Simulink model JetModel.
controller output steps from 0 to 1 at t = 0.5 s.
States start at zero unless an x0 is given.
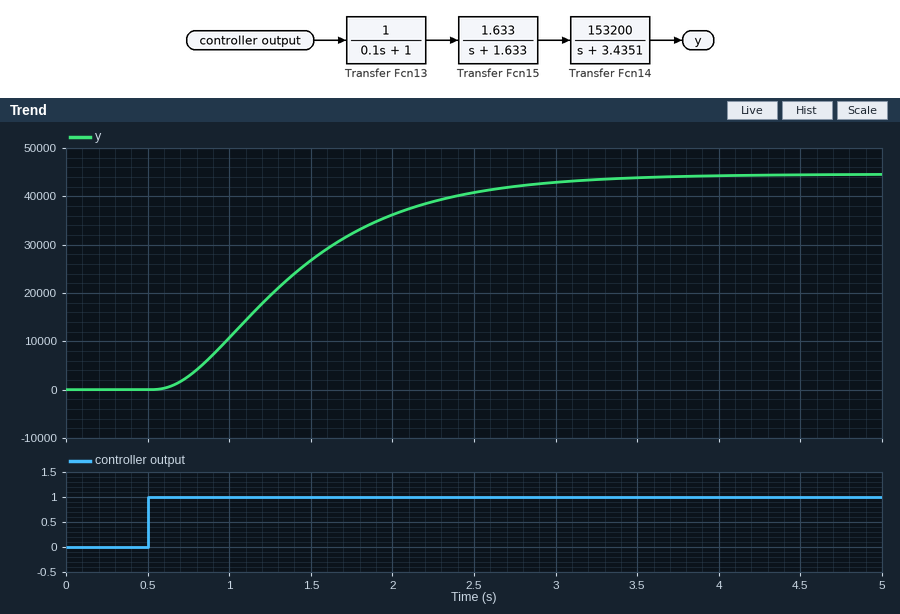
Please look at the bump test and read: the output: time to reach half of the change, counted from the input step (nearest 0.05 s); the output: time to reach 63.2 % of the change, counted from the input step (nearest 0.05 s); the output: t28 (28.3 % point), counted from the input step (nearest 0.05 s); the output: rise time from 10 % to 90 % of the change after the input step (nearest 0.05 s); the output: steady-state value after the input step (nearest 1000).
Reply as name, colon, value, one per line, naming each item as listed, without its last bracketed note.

the output: time to reach half of the change, counted from the input step: 0.85 s
the output: time to reach 63.2 % of the change, counted from the input step: 1.05 s
the output: t28 (28.3 % point), counted from the input step: 0.55 s
the output: rise time from 10 % to 90 % of the change after the input step: 1.60 s
the output: steady-state value after the input step: 45000
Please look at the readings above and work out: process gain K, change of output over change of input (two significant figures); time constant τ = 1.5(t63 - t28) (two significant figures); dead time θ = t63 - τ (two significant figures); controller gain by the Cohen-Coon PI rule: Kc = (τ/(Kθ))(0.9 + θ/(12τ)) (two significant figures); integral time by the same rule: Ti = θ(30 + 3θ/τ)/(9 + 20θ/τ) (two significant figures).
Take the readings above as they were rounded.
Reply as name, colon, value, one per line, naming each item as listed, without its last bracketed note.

process gain K, change of output over change of input: 45000
time constant τ = 1.5(t63 - t28): 0.75 s
dead time θ = t63 - τ: 0.30 s
controller gain by the Cohen-Coon PI rule: Kc = (τ/(Kθ))(0.9 + θ/(12τ)): 0.000052
integral time by the same rule: Ti = θ(30 + 3θ/τ)/(9 + 20θ/τ): 0.55 s
